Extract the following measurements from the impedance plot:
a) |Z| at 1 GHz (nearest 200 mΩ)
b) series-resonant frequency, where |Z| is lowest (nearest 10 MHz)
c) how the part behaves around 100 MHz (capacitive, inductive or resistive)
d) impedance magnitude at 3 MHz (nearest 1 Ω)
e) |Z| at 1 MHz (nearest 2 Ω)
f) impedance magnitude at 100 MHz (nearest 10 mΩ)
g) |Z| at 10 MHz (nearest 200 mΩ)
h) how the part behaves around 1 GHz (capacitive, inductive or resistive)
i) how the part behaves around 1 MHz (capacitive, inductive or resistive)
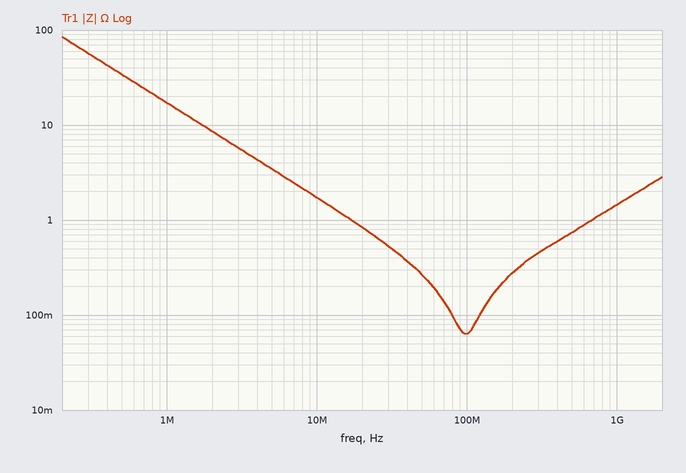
1.4 Ω
100 MHz
resistive
6 Ω
18 Ω
60 mΩ
1.8 Ω
inductive
capacitive
